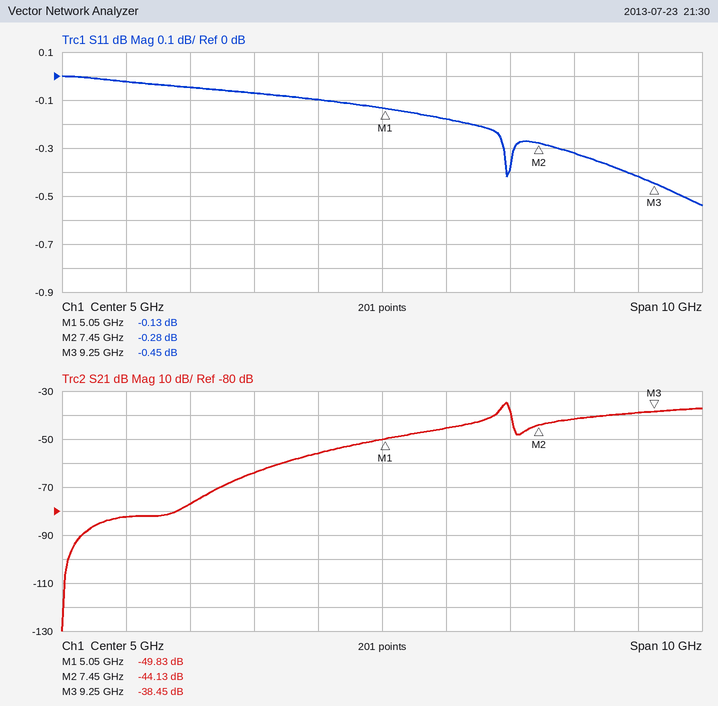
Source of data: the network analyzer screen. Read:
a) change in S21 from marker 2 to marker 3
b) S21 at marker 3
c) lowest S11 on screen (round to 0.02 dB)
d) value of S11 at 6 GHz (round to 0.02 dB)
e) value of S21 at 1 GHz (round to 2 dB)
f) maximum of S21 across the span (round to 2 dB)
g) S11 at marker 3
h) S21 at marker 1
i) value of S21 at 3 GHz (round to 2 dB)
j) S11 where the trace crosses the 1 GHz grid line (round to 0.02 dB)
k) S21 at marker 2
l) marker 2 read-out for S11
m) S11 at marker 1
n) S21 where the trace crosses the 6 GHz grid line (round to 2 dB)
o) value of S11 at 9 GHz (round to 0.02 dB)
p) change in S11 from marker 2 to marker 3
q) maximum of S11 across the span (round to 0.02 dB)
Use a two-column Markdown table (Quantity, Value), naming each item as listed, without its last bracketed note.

| Quantity | Value |
|---|---|
| change in S21 from marker 2 to marker 3 | 5.68 dB |
| S21 at marker 3 | -38.45 dB |
| lowest S11 on screen | -0.54 dB |
| value of S11 at 6 GHz | -0.18 dB |
| value of S21 at 1 GHz | -82 dB |
| maximum of S21 across the span | -34 dB |
| S11 at marker 3 | -0.45 dB |
| S21 at marker 1 | -49.83 dB |
| value of S21 at 3 GHz | -64 dB |
| S11 where the trace crosses the 1 GHz grid line | -0.02 dB |
| S21 at marker 2 | -44.13 dB |
| marker 2 read-out for S11 | -0.28 dB |
| S11 at marker 1 | -0.13 dB |
| S21 where the trace crosses the 6 GHz grid line | -46 dB |
| value of S11 at 9 GHz | -0.42 dB |
| change in S11 from marker 2 to marker 3 | -0.17 dB |
| maximum of S11 across the span | 0.00 dB |
